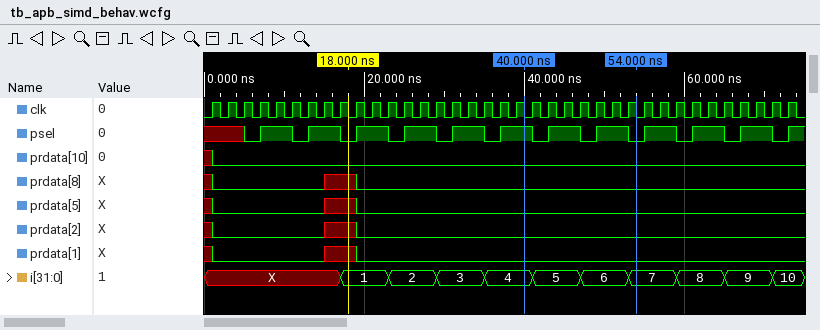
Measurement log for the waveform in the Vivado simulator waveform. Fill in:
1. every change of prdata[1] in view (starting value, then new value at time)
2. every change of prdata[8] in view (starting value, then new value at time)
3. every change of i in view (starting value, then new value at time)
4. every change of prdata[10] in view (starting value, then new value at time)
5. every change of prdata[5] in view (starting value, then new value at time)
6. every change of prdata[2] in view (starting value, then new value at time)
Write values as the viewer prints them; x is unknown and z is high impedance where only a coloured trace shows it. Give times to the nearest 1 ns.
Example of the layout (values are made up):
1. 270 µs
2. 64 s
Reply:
1. x, 0 at 1 ns, x at 15 ns, 0 at 19 ns
2. x, 0 at 1 ns, x at 15 ns, 0 at 19 ns
3. X, 1 at 17 ns, 2 at 23 ns, 3 at 29 ns, 4 at 35 ns, 5 at 41 ns, 6 at 47 ns, 7 at 53 ns, 8 at 59 ns, 9 at 65 ns, 10 at 71 ns
4. x, 0 at 1 ns
5. x, 0 at 1 ns, x at 15 ns, 0 at 19 ns
6. x, 0 at 1 ns, x at 15 ns, 0 at 19 ns
